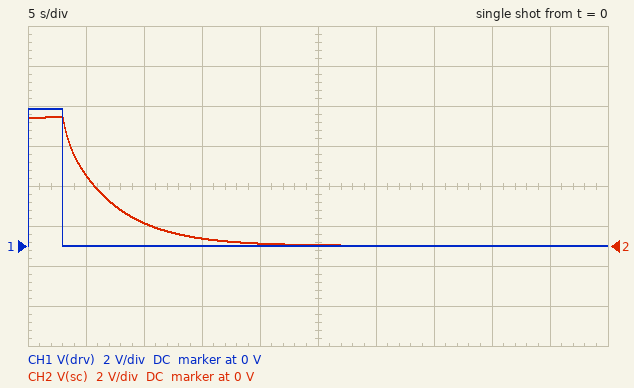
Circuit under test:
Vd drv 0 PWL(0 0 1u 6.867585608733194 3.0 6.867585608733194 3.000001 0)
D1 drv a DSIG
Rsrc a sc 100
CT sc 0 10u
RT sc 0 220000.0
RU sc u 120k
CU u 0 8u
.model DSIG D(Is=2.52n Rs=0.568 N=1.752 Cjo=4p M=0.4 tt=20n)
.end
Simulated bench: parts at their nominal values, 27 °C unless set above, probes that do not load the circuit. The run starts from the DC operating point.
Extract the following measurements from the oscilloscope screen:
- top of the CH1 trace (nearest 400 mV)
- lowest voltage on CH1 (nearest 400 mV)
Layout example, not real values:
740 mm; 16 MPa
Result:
6.8 V; 0 V
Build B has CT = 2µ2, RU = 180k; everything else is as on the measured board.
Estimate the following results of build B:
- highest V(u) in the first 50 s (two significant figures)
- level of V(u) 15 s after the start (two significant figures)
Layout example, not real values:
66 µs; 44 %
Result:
5.6 V; 190 mV
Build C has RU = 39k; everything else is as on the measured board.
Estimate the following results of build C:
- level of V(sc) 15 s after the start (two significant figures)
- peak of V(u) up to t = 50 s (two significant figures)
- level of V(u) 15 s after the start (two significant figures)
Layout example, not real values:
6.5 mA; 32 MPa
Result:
330 mV; 6.4 V; 360 mV
